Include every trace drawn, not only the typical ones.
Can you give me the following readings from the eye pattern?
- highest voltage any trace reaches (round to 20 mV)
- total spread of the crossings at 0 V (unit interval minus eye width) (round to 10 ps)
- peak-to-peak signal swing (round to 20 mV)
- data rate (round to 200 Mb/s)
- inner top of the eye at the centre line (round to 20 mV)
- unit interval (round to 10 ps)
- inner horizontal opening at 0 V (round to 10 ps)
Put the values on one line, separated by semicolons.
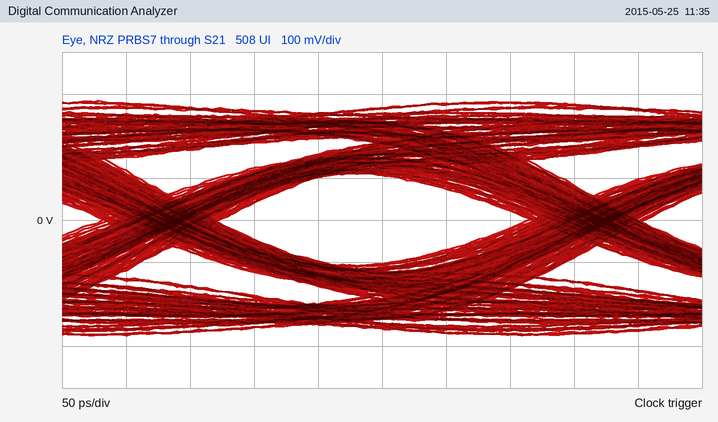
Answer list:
280 mV; 90 ps; 560 mV; 3.0 Gb/s; 100 mV; 330 ps; 240 ps
